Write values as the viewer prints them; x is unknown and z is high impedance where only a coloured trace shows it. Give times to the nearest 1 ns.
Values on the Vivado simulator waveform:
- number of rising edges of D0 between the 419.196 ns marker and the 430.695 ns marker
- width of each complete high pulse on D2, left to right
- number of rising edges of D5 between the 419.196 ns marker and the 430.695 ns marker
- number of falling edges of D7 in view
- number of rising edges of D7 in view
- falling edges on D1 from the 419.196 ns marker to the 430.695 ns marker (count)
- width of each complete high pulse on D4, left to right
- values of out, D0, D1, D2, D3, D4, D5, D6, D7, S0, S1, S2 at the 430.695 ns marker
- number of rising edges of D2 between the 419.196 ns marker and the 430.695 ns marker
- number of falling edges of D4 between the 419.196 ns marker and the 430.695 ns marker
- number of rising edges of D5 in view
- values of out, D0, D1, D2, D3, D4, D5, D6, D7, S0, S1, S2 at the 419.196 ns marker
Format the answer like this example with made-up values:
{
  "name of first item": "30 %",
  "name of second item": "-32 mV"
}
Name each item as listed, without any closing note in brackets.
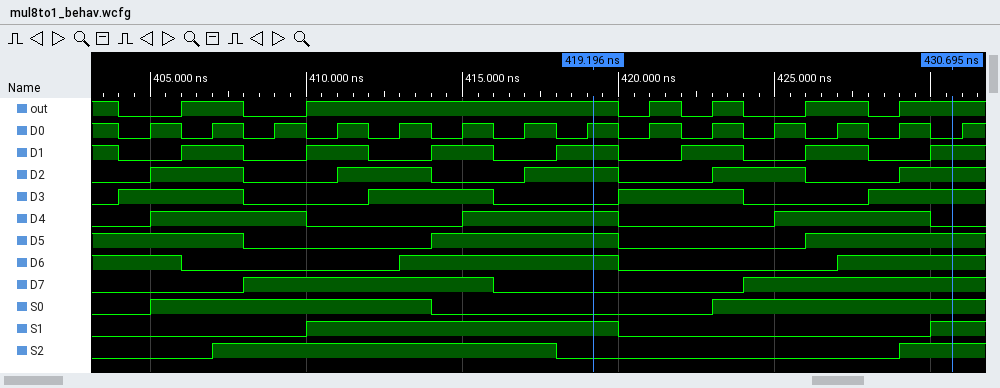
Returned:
{
  "number of rising edges of D0 between the 419.196 ns marker and the 430.695 ns marker": "5",
  "width of each complete high pulse on D2, left to right": "3 ns, 3 ns, 3 ns, 3 ns",
  "number of rising edges of D5 between the 419.196 ns marker and the 430.695 ns marker": "1",
  "number of falling edges of D7 in view": "1",
  "number of rising edges of D7 in view": "2",
  "falling edges on D1 from the 419.196 ns marker to the 430.695 ns marker": "3",
  "width of each complete high pulse on D4, left to right": "5 ns, 5 ns, 5 ns",
  "values of out, D0, D1, D2, D3, D4, D5, D6, D7, S0, S1, S2 at the 430.695 ns marker": "out=1, D0=0, D1=1, D2=1, D3=1, D4=0, D5=1, D6=1, D7=1, S0=1, S1=1, S2=1",
  "number of rising edges of D2 between the 419.196 ns marker and the 430.695 ns marker": "2",
  "number of falling edges of D4 between the 419.196 ns marker and the 430.695 ns marker": "2",
  "number of rising edges of D5 in view": "2",
  "values of out, D0, D1, D2, D3, D4, D5, D6, D7, S0, S1, S2 at the 419.196 ns marker": "out=1, D0=1, D1=1, D2=1, D3=0, D4=1, D5=1, D6=1, D7=0, S0=0, S1=1, S2=0"
}
